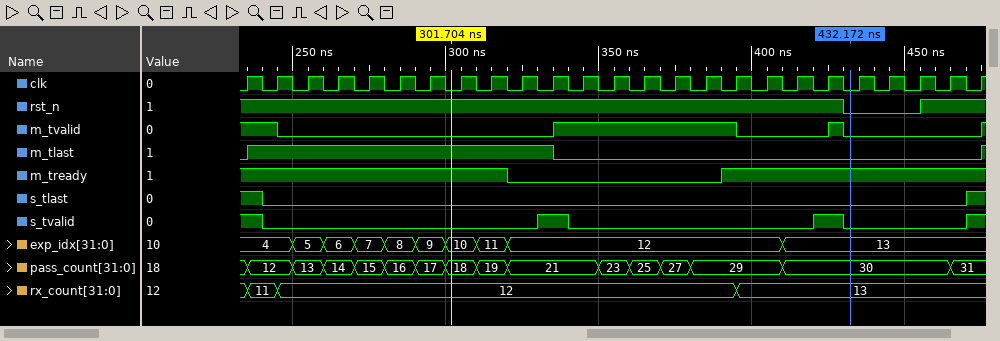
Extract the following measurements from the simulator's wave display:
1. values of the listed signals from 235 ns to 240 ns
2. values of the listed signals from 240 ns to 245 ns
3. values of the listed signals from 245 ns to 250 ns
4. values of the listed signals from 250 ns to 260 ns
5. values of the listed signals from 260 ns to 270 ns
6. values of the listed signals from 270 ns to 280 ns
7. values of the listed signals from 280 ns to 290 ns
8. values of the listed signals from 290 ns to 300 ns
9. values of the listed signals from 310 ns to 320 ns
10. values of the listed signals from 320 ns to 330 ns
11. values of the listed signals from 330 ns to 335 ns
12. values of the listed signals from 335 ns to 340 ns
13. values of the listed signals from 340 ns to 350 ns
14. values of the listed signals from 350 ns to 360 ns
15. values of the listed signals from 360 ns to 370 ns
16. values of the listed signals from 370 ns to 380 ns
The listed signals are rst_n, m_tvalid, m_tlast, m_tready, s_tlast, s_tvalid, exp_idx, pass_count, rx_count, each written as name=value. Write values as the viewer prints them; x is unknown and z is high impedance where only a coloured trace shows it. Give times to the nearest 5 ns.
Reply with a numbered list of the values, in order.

1. rst_n=1, m_tvalid=1, m_tlast=1, m_tready=1, s_tlast=1, s_tvalid=1, exp_idx=4, pass_count=12, rx_count=11
2. rst_n=1, m_tvalid=1, m_tlast=1, m_tready=1, s_tlast=0, s_tvalid=0, exp_idx=4, pass_count=12, rx_count=11
3. rst_n=1, m_tvalid=0, m_tlast=1, m_tready=1, s_tlast=0, s_tvalid=0, exp_idx=4, pass_count=12, rx_count=12
4. rst_n=1, m_tvalid=0, m_tlast=1, m_tready=1, s_tlast=0, s_tvalid=0, exp_idx=5, pass_count=13, rx_count=12
5. rst_n=1, m_tvalid=0, m_tlast=1, m_tready=1, s_tlast=0, s_tvalid=0, exp_idx=6, pass_count=14, rx_count=12
6. rst_n=1, m_tvalid=0, m_tlast=1, m_tready=1, s_tlast=0, s_tvalid=0, exp_idx=7, pass_count=15, rx_count=12
7. rst_n=1, m_tvalid=0, m_tlast=1, m_tready=1, s_tlast=0, s_tvalid=0, exp_idx=8, pass_count=16, rx_count=12
8. rst_n=1, m_tvalid=0, m_tlast=1, m_tready=1, s_tlast=0, s_tvalid=0, exp_idx=9, pass_count=17, rx_count=12
9. rst_n=1, m_tvalid=0, m_tlast=1, m_tready=1, s_tlast=0, s_tvalid=0, exp_idx=11, pass_count=19, rx_count=12
10. rst_n=1, m_tvalid=0, m_tlast=1, m_tready=0, s_tlast=0, s_tvalid=0, exp_idx=12, pass_count=21, rx_count=12
11. rst_n=1, m_tvalid=0, m_tlast=1, m_tready=0, s_tlast=0, s_tvalid=1, exp_idx=12, pass_count=21, rx_count=12
12. rst_n=1, m_tvalid=1, m_tlast=0, m_tready=0, s_tlast=0, s_tvalid=1, exp_idx=12, pass_count=21, rx_count=12
13. rst_n=1, m_tvalid=1, m_tlast=0, m_tready=0, s_tlast=0, s_tvalid=0, exp_idx=12, pass_count=21, rx_count=12
14. rst_n=1, m_tvalid=1, m_tlast=0, m_tready=0, s_tlast=0, s_tvalid=0, exp_idx=12, pass_count=23, rx_count=12
15. rst_n=1, m_tvalid=1, m_tlast=0, m_tready=0, s_tlast=0, s_tvalid=0, exp_idx=12, pass_count=25, rx_count=12
16. rst_n=1, m_tvalid=1, m_tlast=0, m_tready=0, s_tlast=0, s_tvalid=0, exp_idx=12, pass_count=27, rx_count=12
